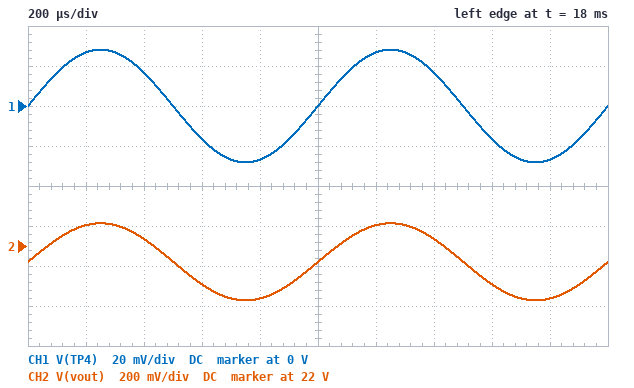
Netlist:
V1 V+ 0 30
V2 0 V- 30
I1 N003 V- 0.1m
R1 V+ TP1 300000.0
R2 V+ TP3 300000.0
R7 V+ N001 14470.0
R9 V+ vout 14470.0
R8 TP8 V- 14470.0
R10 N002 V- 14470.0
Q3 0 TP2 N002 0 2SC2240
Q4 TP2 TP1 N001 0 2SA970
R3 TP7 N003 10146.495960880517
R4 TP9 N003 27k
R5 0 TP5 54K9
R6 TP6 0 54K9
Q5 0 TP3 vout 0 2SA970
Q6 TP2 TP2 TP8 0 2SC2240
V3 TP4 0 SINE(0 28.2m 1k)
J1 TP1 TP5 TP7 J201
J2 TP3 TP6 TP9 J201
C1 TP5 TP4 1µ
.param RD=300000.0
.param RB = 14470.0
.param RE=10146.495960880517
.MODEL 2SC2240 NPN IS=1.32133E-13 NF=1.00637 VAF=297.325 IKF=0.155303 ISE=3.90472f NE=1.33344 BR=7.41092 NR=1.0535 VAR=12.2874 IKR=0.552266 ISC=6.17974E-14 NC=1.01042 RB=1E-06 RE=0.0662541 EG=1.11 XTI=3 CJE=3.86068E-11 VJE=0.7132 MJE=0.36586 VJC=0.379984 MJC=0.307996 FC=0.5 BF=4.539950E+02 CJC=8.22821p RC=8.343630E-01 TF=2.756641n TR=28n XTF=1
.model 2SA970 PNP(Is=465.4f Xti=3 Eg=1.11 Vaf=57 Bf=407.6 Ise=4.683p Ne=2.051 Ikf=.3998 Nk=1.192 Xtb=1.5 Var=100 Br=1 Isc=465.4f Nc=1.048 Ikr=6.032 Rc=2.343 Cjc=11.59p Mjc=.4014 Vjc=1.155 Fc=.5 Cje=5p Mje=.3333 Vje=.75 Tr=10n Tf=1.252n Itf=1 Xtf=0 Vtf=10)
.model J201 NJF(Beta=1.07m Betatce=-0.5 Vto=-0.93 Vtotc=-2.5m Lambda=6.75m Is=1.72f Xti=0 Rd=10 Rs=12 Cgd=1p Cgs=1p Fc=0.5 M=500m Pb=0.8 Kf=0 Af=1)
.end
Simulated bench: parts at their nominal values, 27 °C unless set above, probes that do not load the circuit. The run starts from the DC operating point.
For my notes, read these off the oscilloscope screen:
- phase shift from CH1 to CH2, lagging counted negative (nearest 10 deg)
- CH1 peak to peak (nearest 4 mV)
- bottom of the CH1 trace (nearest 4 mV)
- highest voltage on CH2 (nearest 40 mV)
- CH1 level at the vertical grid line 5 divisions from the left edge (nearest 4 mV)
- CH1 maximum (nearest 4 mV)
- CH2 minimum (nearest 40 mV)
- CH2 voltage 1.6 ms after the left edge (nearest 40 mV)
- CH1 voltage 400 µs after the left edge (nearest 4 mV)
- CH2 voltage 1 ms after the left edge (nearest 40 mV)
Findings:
0 deg
56 mV
-28 mV
22.12 V
0 V
28 mV
21.72 V
21.80 V
16 mV
21.92 V
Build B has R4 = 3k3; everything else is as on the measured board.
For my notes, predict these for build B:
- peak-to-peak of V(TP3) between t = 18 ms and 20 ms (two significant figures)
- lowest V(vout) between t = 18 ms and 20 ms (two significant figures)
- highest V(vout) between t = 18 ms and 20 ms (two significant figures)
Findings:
880 mV
10 V
11 V
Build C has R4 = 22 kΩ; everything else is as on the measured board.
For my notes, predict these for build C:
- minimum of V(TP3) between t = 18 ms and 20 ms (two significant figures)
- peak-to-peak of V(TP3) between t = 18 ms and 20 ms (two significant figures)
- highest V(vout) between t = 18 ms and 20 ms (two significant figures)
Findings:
20 V
440 mV
21 V
